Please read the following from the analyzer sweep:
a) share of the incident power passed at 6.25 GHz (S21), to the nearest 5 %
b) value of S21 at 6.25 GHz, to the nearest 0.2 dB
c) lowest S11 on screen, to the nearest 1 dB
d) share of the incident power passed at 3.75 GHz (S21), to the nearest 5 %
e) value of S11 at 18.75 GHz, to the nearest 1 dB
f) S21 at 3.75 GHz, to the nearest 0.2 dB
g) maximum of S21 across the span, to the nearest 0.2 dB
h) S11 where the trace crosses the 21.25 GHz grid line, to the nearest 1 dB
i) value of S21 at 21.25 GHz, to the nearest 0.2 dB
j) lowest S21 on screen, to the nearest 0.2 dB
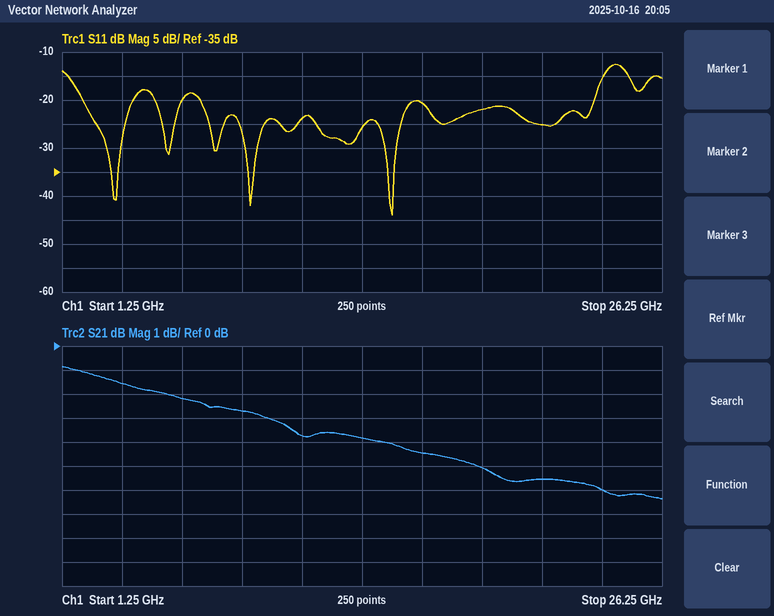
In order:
60 %
-2.2 dB
-44 dB
70 %
-22 dB
-1.6 dB
-0.8 dB
-25 dB
-5.6 dB
-6.4 dB
